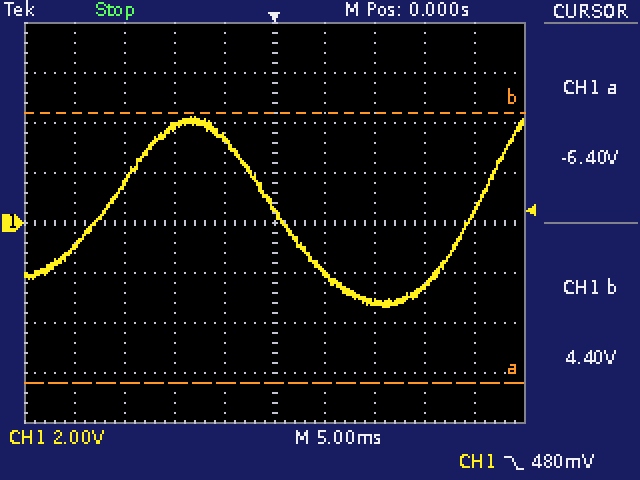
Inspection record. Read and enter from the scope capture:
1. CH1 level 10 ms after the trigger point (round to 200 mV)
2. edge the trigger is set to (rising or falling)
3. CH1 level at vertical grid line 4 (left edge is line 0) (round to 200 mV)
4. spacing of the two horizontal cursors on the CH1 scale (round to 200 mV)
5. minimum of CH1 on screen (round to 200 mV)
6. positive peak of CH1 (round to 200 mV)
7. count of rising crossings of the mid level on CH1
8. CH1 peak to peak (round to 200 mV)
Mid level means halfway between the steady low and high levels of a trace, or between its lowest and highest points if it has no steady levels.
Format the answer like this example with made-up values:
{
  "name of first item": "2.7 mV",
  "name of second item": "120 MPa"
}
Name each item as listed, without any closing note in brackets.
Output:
{
  "CH1 level 10 ms after the trigger point": "-3.2 V",
  "edge the trigger is set to": "falling",
  "CH1 level at vertical grid line 4 (left edge is line 0)": "3.4 V",
  "spacing of the two horizontal cursors on the CH1 scale": "10.8 V",
  "minimum of CH1 on screen": "-3.4 V",
  "positive peak of CH1": "4.2 V",
  "count of rising crossings of the mid level on CH1": "2",
  "CH1 peak to peak": "7.6 V"
}
